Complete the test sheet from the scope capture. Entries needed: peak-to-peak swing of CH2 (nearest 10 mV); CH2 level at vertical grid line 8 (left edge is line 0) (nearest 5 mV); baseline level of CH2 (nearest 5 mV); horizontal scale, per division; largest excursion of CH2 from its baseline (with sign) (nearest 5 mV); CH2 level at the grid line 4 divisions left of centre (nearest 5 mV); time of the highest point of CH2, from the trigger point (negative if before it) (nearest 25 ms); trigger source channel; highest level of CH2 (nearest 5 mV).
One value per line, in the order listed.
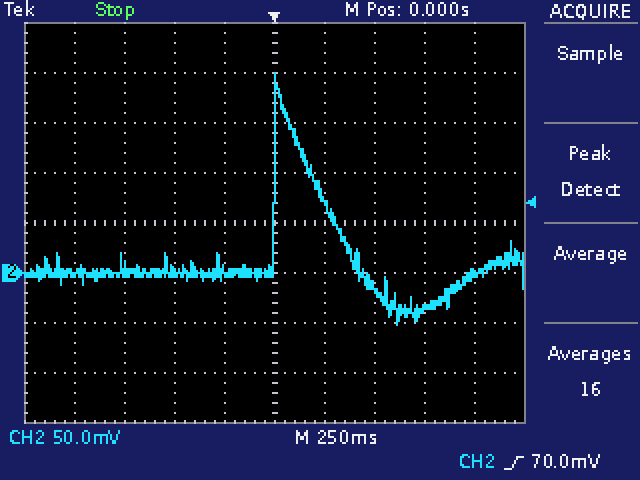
250 mV
-35 mV
0 mV
250 ms
+200 mV
0 mV
0 ms
CH2
200 mV
